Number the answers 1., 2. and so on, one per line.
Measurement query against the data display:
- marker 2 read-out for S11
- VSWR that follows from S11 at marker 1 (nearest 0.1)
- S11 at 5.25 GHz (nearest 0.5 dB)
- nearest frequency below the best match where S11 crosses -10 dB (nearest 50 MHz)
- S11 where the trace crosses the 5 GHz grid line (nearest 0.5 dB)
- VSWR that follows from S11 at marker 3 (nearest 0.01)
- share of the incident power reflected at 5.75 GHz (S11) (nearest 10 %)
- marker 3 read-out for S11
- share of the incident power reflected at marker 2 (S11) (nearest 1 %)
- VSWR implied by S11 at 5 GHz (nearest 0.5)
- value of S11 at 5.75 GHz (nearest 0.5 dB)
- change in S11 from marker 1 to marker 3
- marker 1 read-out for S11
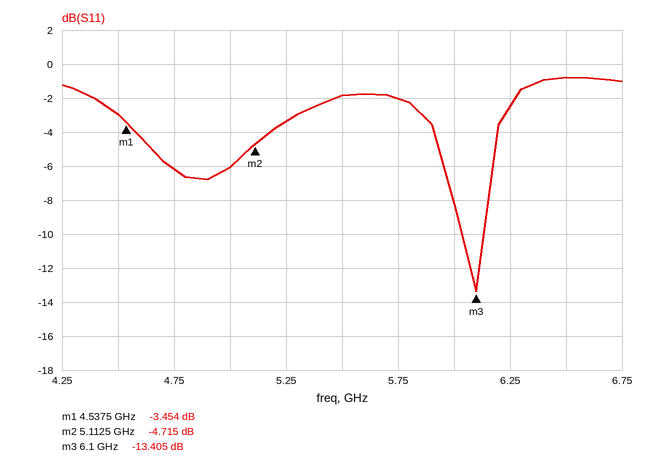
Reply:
1. -4.715 dB
2. 5.1
3. -3.5 dB
4. 6.05 GHz
5. -6.0 dB
6. 1.54
7. 60 %
8. -13.405 dB
9. 34 %
10. 3.0
11. -2.0 dB
12. -9.951 dB
13. -3.454 dB
